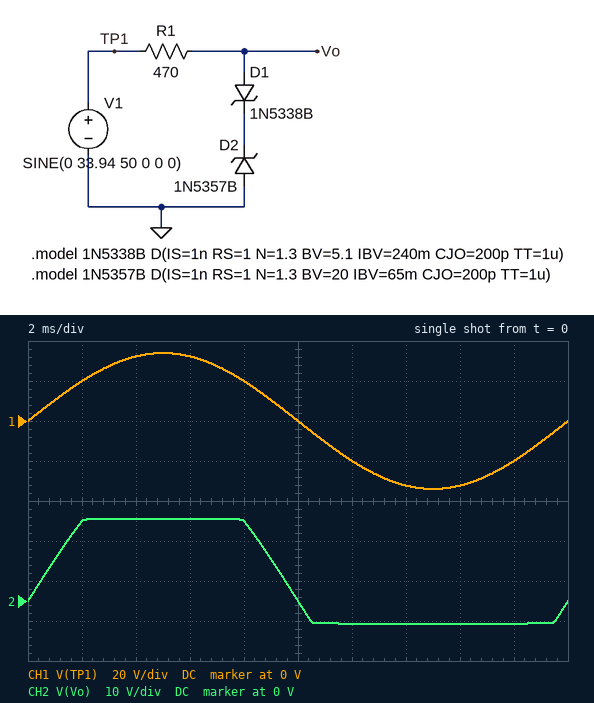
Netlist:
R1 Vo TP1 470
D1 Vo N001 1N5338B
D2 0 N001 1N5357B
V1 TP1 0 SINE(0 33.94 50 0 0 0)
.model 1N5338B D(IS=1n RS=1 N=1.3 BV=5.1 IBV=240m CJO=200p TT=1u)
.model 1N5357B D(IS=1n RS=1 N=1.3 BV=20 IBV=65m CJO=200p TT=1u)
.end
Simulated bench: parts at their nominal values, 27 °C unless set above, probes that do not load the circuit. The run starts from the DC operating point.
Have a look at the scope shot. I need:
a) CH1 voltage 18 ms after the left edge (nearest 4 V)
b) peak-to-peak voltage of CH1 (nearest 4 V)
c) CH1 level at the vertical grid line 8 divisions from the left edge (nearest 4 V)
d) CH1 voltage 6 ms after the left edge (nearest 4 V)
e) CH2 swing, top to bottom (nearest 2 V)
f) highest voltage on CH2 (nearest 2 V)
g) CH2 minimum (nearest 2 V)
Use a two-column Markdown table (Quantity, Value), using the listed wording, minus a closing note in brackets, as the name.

| Quantity | Value |
|---|---|
| CH1 voltage 18 ms after the left edge | -20 V |
| peak-to-peak voltage of CH1 | 68 V |
| CH1 level at the vertical grid line 8 divisions from the left edge | -32 V |
| CH1 voltage 6 ms after the left edge | 32 V |
| CH2 swing, top to bottom | 26 V |
| highest voltage on CH2 | 20 V |
| CH2 minimum | -6 V |
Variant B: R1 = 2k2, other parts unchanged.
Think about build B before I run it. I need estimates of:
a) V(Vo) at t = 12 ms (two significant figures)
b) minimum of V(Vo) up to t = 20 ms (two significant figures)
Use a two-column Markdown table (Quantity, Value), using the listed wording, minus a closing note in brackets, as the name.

| Quantity | Value |
|---|---|
| V(Vo) at t = 12 ms | -5.5 V |
| minimum of V(Vo) up to t = 20 ms | -5.6 V |
